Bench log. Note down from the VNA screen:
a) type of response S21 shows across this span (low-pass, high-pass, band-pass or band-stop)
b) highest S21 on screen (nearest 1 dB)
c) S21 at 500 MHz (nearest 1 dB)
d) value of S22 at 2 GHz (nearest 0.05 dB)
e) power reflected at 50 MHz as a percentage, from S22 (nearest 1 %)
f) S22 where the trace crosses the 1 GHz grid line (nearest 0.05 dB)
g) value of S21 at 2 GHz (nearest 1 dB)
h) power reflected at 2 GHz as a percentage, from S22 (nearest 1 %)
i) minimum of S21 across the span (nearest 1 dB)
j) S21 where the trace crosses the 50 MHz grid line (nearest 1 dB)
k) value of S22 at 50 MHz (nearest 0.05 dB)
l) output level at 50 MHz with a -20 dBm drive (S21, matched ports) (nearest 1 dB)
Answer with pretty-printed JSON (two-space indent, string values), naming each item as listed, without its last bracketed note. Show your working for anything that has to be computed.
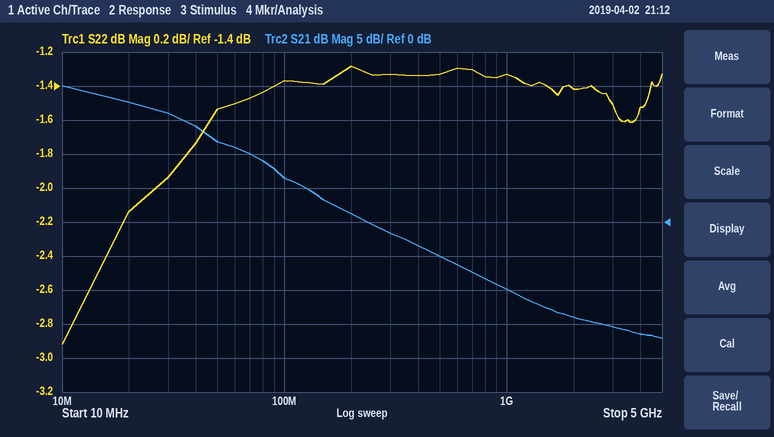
{
  "type of response S21 shows across this span": "low-pass",
  "highest S21 on screen": "20 dB",
  "S21 at 500 MHz": "-5 dB",
  "value of S22 at 2 GHz": "-1.40 dB",
  "power reflected at 50 MHz as a percentage, from S22": "10^(-1.55/10) ≈ 70 %",
  "S22 where the trace crosses the 1 GHz grid line": "-1.35 dB",
  "value of S21 at 2 GHz": "-14 dB",
  "power reflected at 2 GHz as a percentage, from S22": "10^(-1.4/10) ≈ 72 %",
  "minimum of S21 across the span": "-17 dB",
  "S21 where the trace crosses the 50 MHz grid line": "12 dB",
  "value of S22 at 50 MHz": "-1.55 dB",
  "output level at 50 MHz with a -20 dBm drive (S21, matched ports)": "-20 dBm + (12 dB) = -8 dBm"
}
